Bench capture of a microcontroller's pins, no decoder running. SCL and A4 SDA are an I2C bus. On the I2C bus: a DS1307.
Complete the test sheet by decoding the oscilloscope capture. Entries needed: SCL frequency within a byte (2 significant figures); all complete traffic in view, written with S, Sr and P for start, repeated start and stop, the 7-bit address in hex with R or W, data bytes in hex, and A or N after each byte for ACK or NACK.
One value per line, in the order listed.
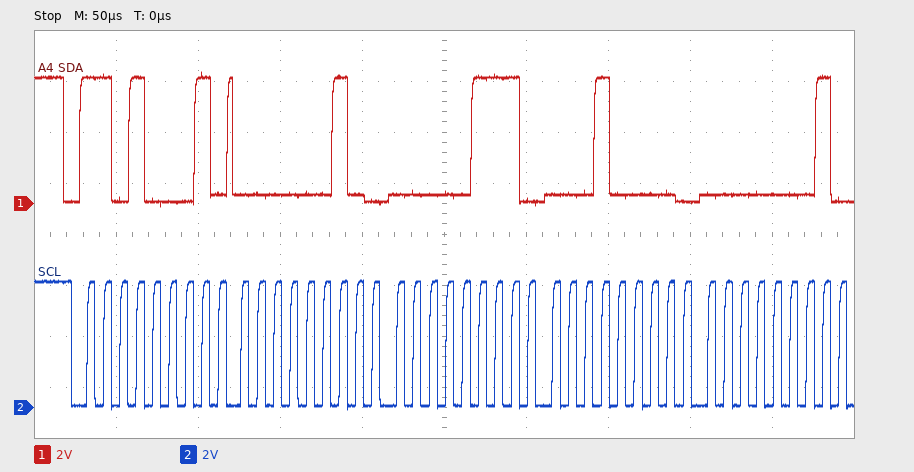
100 kHz
S 68R A 02 A 07 A 10 A 01 A
